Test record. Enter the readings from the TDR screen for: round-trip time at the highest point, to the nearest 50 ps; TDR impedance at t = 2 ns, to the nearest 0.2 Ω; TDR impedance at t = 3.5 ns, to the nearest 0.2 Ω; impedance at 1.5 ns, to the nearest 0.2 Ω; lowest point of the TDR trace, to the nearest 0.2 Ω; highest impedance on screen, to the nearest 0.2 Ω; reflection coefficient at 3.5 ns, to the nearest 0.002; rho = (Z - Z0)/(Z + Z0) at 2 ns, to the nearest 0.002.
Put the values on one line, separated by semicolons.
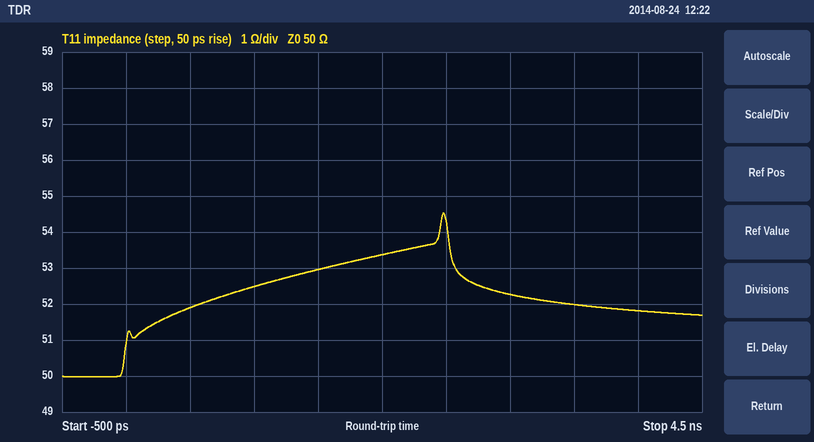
2.50 ns; 53.4 Ω; 52.0 Ω; 53.0 Ω; 50.0 Ω; 54.6 Ω; +0.020; +0.032
